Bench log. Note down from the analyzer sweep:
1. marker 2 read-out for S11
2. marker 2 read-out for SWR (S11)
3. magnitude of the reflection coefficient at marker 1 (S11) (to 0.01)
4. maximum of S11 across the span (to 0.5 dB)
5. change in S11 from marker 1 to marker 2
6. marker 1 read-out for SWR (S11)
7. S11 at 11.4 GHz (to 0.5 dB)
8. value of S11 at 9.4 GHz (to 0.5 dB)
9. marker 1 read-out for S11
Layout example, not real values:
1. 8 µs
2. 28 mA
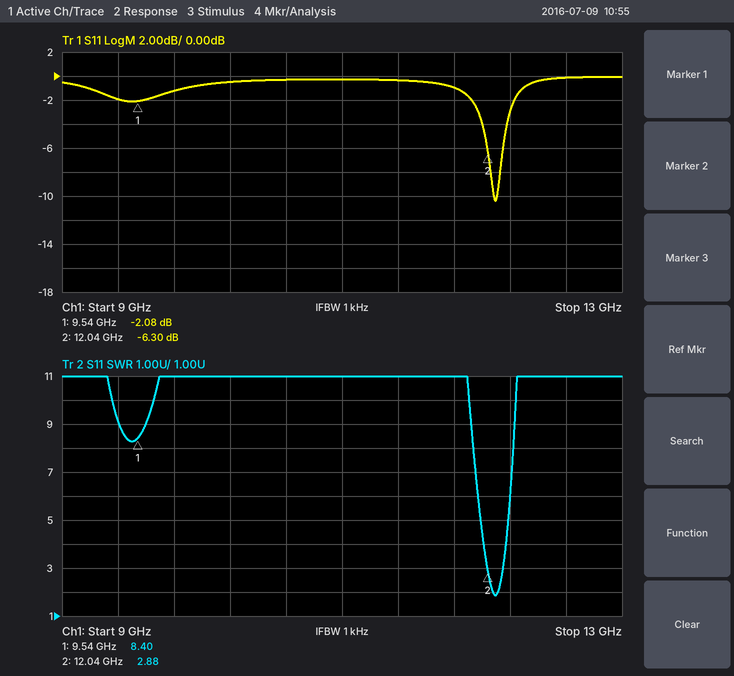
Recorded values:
1. -6.30 dB
2. 2.88
3. 0.79
4. 0.0 dB
5. -4.22 dB
6. 8.40
7. -0.5 dB
8. -2.0 dB
9. -2.08 dB
